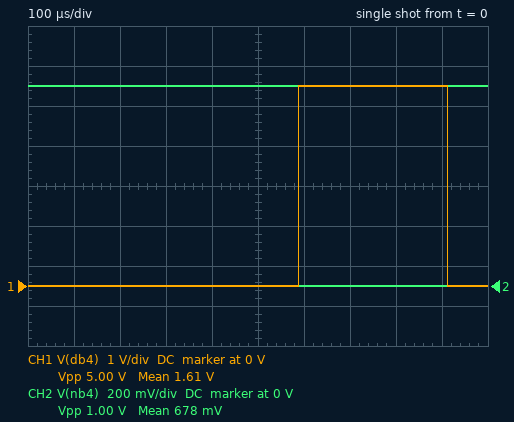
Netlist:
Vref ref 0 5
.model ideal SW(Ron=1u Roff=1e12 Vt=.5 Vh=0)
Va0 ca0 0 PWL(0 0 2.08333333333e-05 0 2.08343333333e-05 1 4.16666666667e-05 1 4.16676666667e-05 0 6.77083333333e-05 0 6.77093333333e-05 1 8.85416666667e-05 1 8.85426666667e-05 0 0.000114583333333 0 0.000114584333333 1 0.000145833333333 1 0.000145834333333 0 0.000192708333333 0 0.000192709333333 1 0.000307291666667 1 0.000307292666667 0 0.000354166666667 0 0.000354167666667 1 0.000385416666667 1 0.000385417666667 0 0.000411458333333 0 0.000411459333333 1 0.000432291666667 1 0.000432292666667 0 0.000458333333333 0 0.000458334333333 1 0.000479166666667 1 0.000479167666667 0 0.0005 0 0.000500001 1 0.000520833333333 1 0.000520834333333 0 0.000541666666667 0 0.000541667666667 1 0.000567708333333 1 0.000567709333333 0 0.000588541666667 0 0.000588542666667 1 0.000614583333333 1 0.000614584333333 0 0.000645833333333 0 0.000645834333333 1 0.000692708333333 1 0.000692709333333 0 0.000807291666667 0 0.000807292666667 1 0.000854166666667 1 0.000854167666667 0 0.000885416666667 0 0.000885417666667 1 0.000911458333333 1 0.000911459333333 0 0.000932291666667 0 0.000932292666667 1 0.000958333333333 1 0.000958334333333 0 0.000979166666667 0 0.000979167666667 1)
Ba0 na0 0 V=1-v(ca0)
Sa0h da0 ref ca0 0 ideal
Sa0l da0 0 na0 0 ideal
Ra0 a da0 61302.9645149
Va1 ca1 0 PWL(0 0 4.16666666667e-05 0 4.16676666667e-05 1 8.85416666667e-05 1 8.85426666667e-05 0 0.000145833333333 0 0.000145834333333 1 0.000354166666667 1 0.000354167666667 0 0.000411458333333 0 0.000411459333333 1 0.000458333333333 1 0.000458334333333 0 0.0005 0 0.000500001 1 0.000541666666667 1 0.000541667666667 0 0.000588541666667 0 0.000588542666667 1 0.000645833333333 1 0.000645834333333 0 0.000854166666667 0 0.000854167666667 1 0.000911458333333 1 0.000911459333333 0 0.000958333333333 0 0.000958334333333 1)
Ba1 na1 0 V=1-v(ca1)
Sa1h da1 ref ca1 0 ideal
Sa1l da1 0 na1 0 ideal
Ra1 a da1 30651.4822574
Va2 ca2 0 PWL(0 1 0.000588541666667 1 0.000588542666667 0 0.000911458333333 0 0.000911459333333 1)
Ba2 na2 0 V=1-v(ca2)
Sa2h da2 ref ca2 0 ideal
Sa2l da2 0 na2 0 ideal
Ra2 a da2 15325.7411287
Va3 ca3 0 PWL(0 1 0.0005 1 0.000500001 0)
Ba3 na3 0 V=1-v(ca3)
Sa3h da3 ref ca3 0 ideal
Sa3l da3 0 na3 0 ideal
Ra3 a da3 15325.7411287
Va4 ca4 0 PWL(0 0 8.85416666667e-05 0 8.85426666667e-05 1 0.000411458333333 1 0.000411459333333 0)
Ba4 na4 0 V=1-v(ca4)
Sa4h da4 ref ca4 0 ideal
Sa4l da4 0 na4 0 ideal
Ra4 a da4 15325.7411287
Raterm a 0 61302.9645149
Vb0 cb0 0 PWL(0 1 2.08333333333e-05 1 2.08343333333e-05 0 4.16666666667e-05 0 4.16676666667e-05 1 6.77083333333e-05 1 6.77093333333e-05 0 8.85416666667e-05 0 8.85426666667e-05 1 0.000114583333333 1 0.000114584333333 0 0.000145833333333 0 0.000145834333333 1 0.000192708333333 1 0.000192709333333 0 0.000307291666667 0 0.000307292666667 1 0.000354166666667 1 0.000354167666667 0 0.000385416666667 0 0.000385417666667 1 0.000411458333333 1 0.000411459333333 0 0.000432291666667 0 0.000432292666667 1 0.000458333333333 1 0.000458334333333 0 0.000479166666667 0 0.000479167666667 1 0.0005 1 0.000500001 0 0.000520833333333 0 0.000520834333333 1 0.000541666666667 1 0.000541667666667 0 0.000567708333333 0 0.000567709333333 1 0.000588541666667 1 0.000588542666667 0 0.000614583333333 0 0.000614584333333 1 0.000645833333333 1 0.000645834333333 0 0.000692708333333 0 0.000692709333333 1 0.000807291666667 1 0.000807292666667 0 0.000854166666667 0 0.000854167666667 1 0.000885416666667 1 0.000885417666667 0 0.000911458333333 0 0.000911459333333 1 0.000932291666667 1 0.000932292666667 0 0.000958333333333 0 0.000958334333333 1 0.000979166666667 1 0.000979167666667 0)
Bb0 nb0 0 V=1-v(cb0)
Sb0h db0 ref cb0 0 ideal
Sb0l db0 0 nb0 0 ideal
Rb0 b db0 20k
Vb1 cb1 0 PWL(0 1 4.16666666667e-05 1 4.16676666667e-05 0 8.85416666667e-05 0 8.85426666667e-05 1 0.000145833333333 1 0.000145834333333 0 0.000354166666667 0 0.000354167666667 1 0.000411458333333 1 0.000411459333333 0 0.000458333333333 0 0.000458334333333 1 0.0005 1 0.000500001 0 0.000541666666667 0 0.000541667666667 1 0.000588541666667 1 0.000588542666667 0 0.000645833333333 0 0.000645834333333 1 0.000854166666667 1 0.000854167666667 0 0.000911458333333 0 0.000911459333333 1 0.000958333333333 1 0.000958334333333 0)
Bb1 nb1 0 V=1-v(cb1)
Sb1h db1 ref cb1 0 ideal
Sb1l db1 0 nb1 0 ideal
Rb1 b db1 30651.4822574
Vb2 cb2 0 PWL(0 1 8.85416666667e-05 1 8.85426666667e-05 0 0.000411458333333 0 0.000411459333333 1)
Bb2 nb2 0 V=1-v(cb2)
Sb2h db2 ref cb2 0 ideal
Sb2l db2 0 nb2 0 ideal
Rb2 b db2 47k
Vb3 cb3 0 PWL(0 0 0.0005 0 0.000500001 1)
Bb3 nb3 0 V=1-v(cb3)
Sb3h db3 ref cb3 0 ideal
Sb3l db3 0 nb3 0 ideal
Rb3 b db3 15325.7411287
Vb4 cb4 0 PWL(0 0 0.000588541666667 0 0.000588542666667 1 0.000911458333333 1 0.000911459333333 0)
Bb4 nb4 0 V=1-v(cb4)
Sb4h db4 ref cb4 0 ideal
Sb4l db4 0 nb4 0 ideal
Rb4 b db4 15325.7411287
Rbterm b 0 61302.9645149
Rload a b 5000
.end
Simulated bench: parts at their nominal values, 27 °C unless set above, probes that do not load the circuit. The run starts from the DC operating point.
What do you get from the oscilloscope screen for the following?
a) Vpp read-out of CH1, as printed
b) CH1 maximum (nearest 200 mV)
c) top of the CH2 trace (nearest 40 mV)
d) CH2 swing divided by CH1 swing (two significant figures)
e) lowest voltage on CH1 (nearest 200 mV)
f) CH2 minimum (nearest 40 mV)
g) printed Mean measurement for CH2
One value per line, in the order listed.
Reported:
5.00 V
5.0 V
1.00 V
0.20
0 V
0 V
678 mV
